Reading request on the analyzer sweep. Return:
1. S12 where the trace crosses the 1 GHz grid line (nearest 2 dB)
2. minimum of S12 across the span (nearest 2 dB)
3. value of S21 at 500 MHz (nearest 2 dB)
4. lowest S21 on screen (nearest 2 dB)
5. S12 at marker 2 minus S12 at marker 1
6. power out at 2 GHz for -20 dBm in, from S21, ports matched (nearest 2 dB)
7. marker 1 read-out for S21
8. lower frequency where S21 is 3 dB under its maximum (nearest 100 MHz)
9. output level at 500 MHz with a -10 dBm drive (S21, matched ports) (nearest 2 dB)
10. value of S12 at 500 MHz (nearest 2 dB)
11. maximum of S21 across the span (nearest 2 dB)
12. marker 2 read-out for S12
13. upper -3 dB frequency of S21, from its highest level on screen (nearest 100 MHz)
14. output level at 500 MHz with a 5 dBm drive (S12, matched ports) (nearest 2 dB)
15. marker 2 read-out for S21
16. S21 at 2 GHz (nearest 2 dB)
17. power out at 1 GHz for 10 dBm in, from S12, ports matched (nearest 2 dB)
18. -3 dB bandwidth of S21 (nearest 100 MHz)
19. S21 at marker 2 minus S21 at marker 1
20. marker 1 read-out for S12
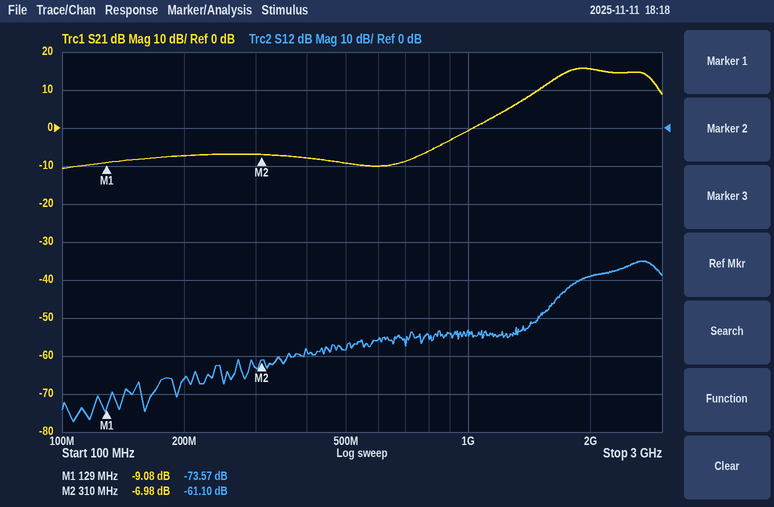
-54 dB
-78 dB
-10 dB
-10 dB
12.47 dB
-4 dBm
-9.08 dB
1.6 GHz
-20 dBm
-58 dB
16 dB
-61.10 dB
2.8 GHz
-54 dBm
-6.98 dB
16 dB
-44 dBm
1.2 GHz
2.10 dB
-73.57 dB
